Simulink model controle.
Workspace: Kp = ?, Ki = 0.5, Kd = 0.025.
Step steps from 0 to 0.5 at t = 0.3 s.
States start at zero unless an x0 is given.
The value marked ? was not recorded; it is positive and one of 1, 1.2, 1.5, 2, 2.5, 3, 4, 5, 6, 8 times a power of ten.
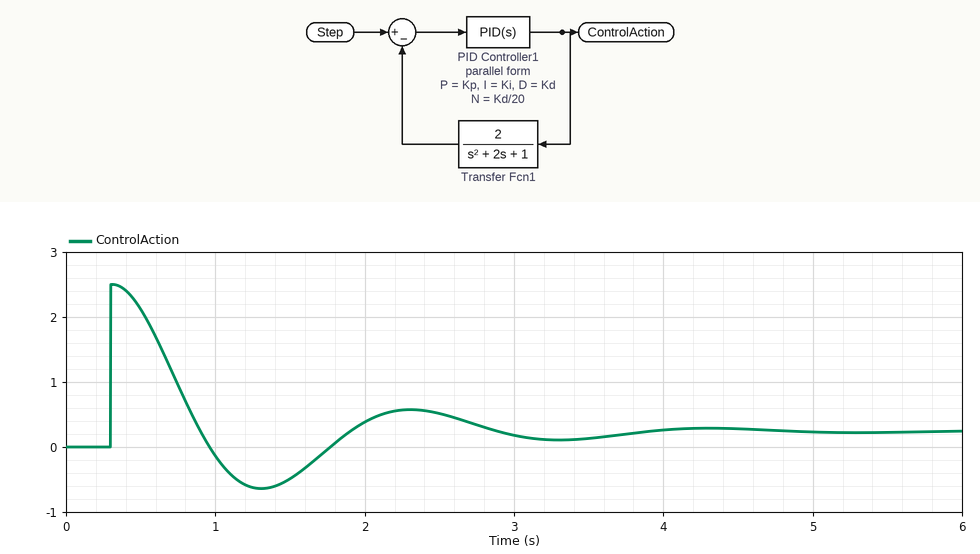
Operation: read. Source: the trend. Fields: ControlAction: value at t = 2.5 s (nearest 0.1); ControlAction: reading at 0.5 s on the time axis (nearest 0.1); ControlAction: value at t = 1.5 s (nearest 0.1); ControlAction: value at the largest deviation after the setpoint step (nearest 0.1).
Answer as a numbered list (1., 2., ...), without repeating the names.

1. 0.5
2. 2.1
3. -0.5
4. 2.5
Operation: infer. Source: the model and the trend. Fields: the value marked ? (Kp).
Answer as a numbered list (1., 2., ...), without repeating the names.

1. 5
